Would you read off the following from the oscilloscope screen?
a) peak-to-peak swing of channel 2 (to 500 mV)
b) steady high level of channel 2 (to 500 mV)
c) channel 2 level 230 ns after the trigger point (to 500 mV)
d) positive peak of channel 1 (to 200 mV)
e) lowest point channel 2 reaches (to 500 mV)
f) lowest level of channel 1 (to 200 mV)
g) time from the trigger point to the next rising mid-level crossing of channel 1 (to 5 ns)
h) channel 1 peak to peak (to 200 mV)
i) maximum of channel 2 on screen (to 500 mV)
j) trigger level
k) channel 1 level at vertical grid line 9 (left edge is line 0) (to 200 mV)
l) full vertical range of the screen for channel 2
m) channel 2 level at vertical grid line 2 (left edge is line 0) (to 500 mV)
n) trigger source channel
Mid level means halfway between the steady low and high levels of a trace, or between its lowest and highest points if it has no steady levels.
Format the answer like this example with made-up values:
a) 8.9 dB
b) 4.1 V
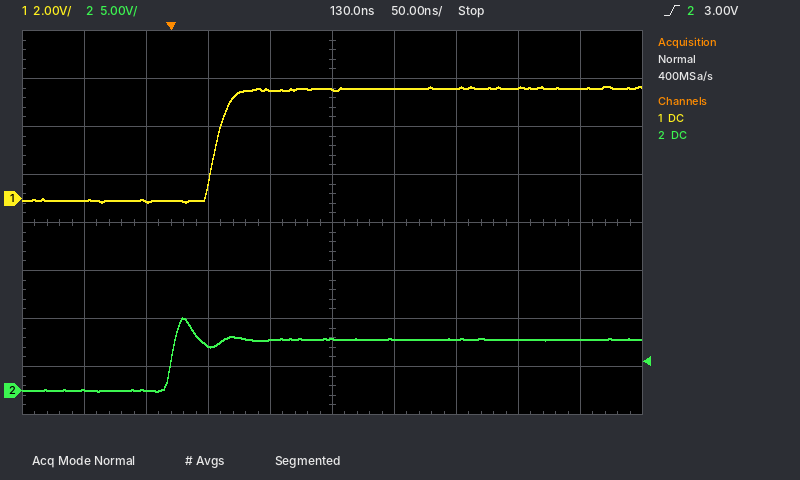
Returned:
a) 7.5 V
b) 5.5 V
c) 5.5 V
d) 4.6 V
e) 0.0 V
f) -200 mV
g) 35 ns
h) 4.8 V
i) 7.5 V
j) 3.00 V
k) 4.6 V
l) 40 V
m) 0.0 V
n) channel 2
